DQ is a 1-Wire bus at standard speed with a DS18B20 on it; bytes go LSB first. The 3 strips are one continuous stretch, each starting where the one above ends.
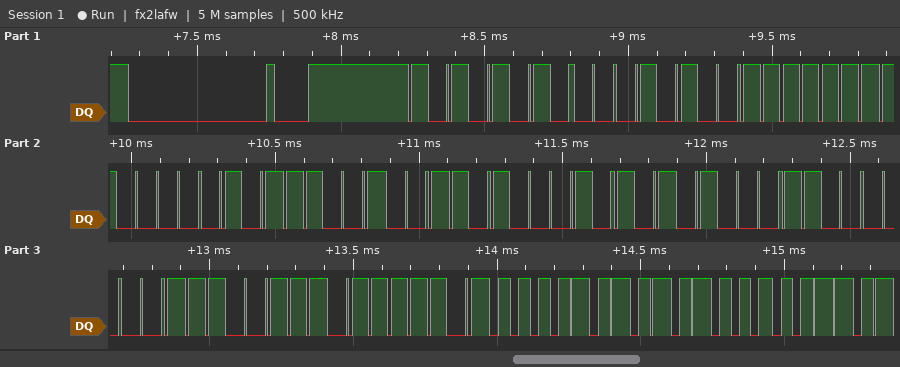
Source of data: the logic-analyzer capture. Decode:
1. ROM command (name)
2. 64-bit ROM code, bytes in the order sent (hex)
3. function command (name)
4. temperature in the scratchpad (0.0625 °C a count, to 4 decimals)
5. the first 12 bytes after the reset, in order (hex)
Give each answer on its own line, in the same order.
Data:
Match ROM
28 FF A0 93 45 15 03 E7
Read Scratchpad
85.0000 °C
55 28 FF A0 93 45 15 03 E7 BE 50 05
